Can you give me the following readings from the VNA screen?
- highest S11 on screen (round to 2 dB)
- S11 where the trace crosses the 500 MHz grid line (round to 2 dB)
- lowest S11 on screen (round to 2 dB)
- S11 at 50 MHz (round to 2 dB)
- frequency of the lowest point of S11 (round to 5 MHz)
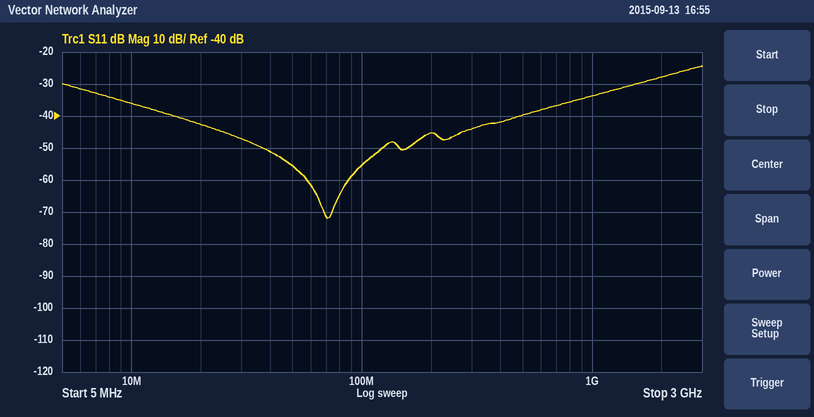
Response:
-24 dB
-40 dB
-72 dB
-56 dB
70 MHz
